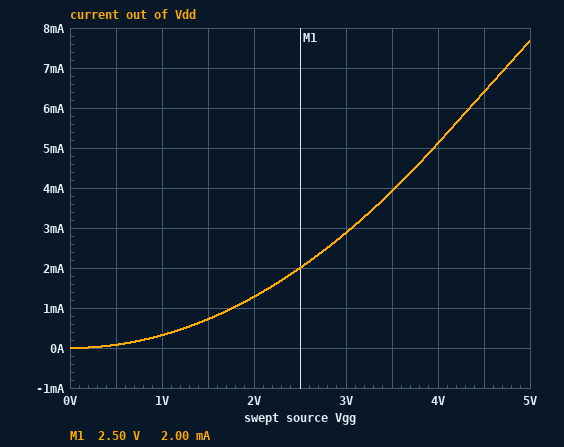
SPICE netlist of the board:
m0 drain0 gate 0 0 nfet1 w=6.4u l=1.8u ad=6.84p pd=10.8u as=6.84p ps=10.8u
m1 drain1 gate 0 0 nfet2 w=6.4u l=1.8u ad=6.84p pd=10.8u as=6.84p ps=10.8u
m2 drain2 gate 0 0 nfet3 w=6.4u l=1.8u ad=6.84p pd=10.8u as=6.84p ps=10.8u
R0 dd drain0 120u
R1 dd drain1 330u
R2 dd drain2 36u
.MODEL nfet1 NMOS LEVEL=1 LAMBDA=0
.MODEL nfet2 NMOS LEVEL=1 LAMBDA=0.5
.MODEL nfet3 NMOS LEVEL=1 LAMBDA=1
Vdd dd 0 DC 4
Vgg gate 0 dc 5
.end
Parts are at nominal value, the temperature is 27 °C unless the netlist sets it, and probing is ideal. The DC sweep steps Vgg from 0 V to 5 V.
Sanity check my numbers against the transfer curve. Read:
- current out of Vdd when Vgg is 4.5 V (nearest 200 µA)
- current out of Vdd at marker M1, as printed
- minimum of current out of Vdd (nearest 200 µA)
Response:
6.4 mA
2.00 mA
0 A
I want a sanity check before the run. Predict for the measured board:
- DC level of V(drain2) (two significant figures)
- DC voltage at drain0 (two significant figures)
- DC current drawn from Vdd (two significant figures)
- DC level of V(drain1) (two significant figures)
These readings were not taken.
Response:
4.0 V
4.0 V
7.7 mA
4.0 V
